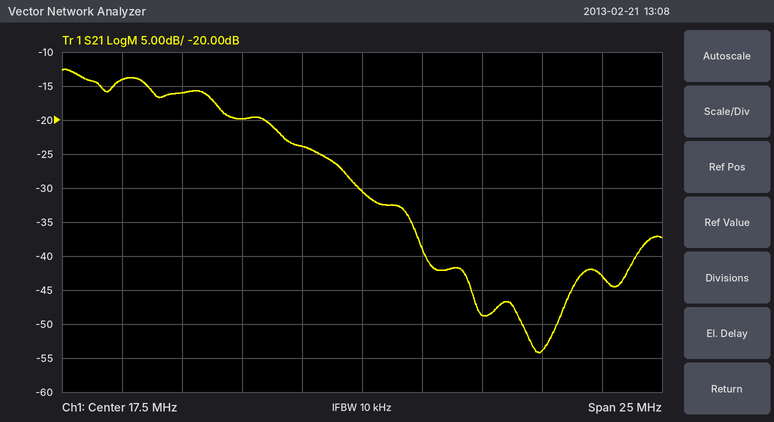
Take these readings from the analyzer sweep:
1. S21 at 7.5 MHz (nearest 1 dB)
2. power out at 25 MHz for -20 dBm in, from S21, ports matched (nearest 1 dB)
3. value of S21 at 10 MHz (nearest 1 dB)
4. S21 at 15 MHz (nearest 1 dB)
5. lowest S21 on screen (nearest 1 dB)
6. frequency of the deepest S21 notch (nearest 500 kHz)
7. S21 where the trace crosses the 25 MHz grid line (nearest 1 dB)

-14 dB
-74 dBm
-16 dB
-24 dB
-54 dB
25.0 MHz
-54 dB
